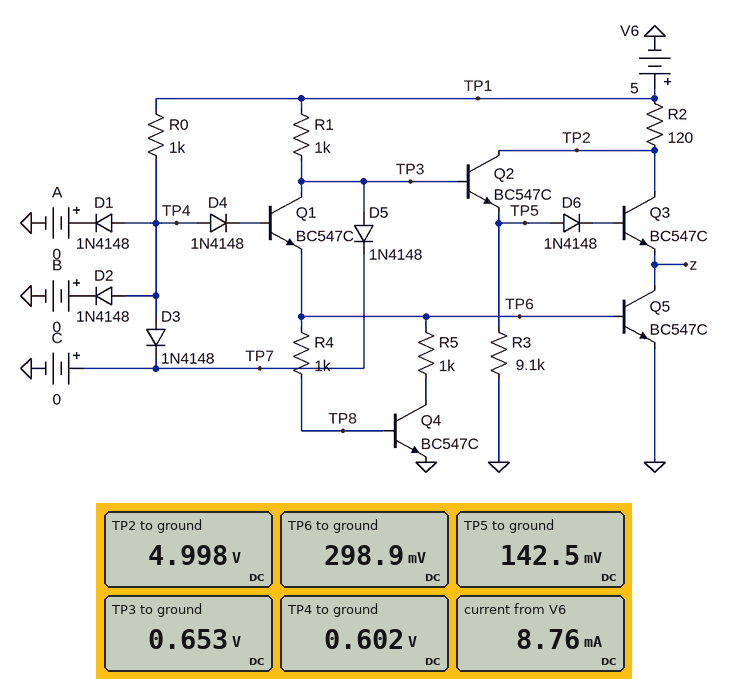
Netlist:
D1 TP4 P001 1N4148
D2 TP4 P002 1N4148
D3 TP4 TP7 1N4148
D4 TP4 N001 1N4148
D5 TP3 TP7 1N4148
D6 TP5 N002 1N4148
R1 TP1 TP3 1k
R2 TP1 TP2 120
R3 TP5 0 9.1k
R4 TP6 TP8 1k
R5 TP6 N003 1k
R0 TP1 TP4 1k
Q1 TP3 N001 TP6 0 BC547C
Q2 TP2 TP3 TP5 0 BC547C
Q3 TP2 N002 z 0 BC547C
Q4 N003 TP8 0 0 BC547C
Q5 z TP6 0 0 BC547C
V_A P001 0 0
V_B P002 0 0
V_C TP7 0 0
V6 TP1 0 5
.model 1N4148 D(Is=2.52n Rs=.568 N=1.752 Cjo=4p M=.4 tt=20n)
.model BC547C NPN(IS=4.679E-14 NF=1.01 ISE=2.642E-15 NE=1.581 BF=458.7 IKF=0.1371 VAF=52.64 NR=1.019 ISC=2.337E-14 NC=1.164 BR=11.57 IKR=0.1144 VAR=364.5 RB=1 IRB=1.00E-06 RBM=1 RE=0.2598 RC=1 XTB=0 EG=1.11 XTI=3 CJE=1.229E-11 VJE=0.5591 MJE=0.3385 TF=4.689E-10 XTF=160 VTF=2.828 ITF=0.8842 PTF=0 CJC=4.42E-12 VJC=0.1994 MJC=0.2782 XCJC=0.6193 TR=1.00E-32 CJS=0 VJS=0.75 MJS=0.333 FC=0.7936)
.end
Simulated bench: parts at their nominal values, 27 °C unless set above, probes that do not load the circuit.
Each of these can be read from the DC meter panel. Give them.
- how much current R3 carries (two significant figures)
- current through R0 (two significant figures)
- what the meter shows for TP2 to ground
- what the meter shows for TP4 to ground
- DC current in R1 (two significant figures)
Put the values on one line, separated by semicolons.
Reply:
16 µA; 4.4 mA; 4.998 V; 0.602 V; 4.3 mA
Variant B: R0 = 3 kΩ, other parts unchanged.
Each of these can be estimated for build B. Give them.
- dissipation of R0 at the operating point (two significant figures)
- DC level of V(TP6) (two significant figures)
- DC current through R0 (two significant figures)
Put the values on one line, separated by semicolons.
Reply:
6.6 mW; 270 mV; 1.5 mA
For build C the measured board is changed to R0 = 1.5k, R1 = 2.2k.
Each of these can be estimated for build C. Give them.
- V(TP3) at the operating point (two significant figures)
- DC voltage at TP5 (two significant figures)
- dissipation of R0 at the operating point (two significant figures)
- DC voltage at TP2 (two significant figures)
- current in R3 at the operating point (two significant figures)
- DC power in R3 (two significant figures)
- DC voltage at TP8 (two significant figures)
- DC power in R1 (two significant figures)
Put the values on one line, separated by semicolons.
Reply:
620 mV; 110 mV; 13 mW; 5.0 V; 12 µA; 1.4 µW; 290 mV; 8.7 mW
